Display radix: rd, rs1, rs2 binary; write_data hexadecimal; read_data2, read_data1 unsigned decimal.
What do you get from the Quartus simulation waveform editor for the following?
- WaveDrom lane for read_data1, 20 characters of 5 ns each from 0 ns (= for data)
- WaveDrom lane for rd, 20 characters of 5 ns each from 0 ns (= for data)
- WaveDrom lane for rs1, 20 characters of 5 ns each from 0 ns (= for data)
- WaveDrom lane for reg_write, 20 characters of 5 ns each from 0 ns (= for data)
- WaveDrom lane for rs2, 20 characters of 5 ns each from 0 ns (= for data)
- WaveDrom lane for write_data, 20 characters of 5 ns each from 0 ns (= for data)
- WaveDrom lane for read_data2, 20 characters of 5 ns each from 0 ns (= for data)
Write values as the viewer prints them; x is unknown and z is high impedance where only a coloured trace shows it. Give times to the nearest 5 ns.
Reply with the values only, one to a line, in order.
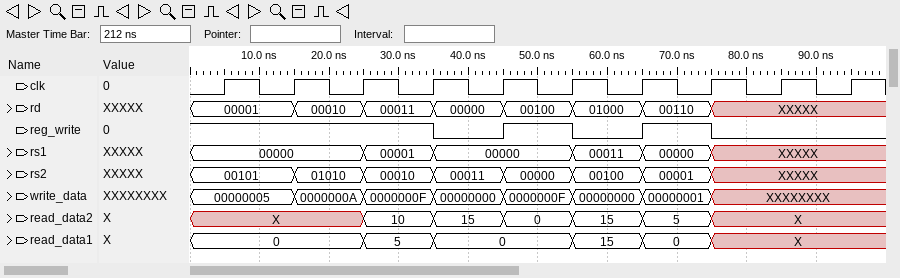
{name: 'read_data1', wave: '=....=.=...=.=.x....', data: '0 5 0 15 0'}
{name: 'rd', wave: '=..=.=.=.=.=.=.x....', data: '00001 00010 00011 00000 00100 01000 00110'}
{name: 'rs1', wave: '=....=.=...=.=.x....', data: '00000 00001 00000 00011 00000'}
{name: 'reg_write', wave: '1......0.1.0.1.0....'}
{name: 'rs2', wave: '=..=.=.=.=.=.=.x....', data: '00101 01010 00010 00011 00000 00100 00001'}
{name: 'write_data', wave: '=..=.=.=.=.=.=.x....', data: '00000005 0000000A 0000000F 00000000 0000000F 00000000 00000001'}
{name: 'read_data2', wave: 'x....=.=.=.=.=.x....', data: '10 15 0 15 5'}
